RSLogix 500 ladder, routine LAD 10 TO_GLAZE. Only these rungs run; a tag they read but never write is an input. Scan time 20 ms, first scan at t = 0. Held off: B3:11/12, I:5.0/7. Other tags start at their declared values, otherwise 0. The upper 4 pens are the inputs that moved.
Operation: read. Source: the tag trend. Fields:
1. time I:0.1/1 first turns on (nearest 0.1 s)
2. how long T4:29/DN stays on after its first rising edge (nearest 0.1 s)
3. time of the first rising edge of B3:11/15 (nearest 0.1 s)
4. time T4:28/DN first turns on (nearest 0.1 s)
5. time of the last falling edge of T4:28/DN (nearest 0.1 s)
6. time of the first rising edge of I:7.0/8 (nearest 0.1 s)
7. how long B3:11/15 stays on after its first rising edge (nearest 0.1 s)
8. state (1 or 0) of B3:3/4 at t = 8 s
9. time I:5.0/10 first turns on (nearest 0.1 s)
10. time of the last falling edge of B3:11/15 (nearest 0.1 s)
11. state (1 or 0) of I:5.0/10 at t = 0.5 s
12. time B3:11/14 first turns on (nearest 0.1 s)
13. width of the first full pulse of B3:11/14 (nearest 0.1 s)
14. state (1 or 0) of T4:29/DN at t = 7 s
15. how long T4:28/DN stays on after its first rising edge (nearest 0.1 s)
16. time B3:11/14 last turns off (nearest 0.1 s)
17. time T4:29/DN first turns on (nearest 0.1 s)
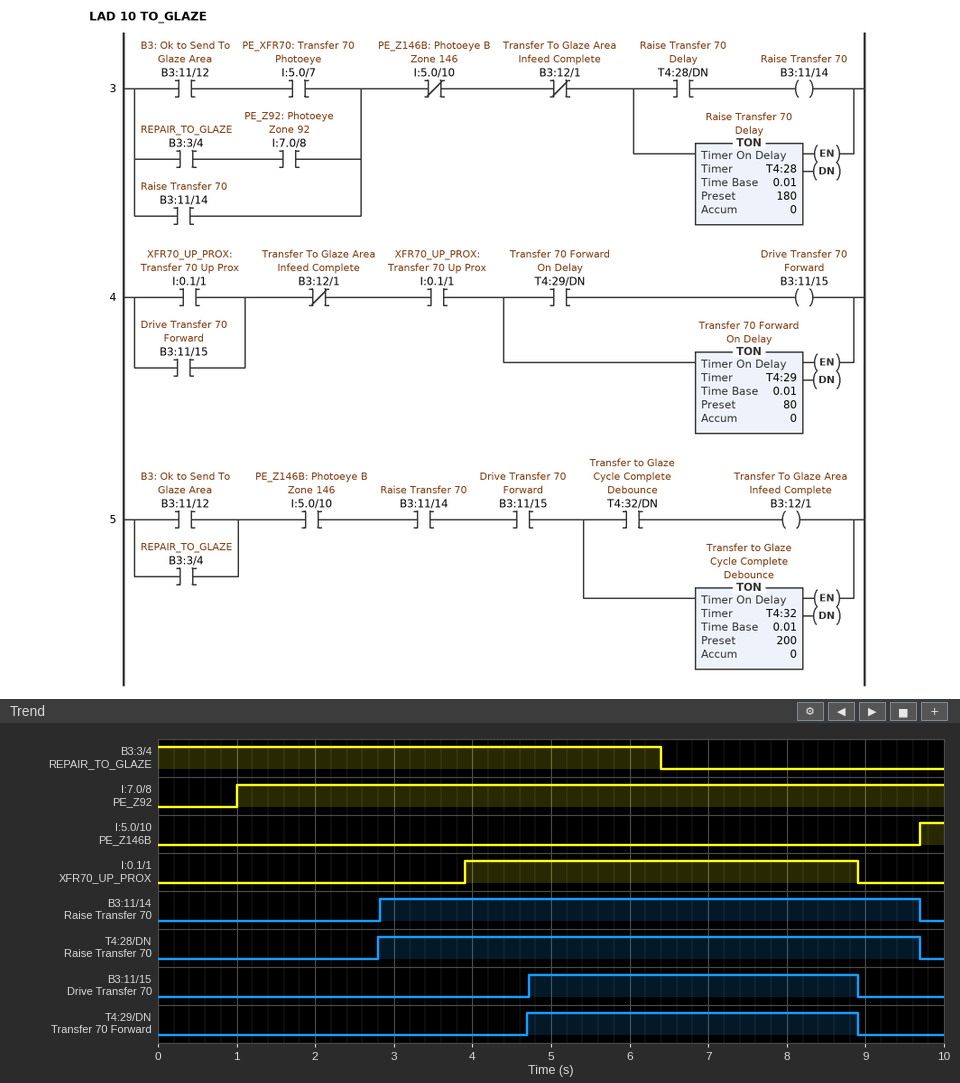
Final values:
3.9 s
4.2 s
4.7 s
2.8 s
9.7 s
1.0 s
4.2 s
0
9.7 s
8.9 s
0
2.8 s
6.9 s
1
6.9 s
9.7 s
4.7 s
